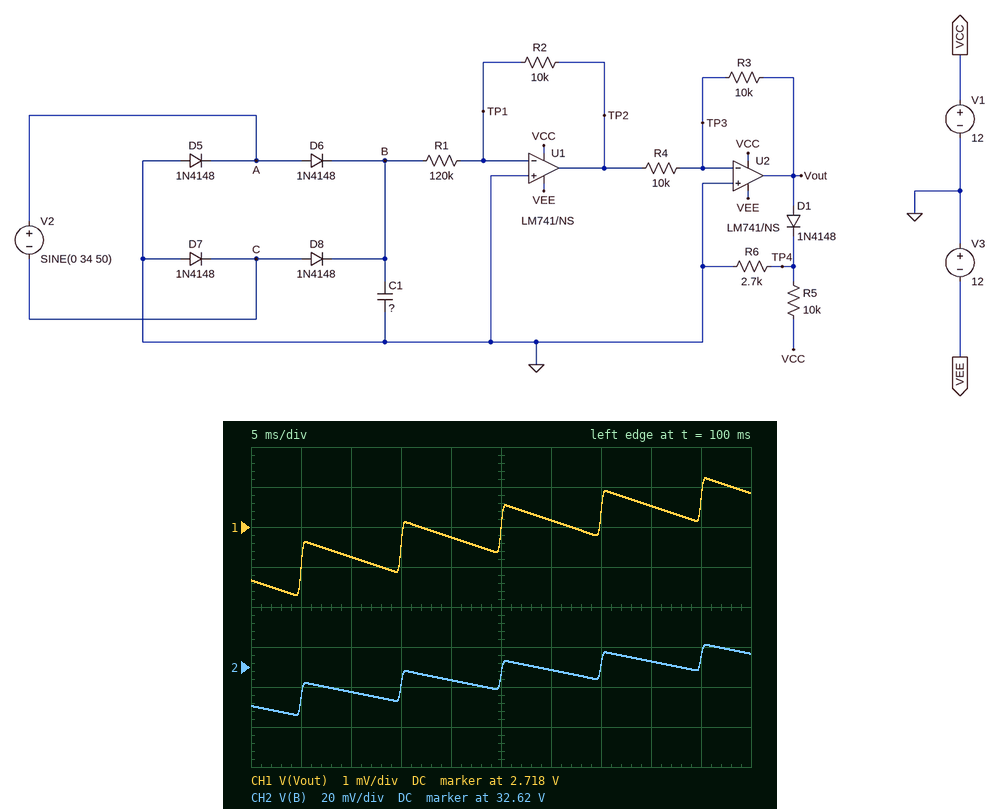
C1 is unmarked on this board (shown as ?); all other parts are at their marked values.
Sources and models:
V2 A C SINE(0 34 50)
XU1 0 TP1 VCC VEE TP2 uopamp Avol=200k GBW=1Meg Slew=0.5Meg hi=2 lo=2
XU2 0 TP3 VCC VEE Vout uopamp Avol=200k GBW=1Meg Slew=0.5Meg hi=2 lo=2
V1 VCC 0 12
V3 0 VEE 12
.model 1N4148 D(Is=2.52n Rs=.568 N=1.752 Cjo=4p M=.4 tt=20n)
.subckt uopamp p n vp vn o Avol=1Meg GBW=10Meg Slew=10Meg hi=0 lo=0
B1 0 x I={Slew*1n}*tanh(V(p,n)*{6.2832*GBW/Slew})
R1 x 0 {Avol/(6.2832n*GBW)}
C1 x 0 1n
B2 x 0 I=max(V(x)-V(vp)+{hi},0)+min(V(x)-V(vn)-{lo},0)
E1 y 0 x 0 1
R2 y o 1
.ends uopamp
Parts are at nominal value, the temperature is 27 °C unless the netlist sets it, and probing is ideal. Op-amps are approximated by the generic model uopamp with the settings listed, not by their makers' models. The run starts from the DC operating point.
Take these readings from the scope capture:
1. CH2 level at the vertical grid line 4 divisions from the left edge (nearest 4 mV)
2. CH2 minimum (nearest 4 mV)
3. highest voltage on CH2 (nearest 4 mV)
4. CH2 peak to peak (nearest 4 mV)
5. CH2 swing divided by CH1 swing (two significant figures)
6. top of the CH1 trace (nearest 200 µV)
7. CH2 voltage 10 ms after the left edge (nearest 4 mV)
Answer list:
32.612 V
32.596 V
32.632 V
36 mV
12
2.7192 V
32.608 V
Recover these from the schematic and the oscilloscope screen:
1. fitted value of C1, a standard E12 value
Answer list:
270 µF
